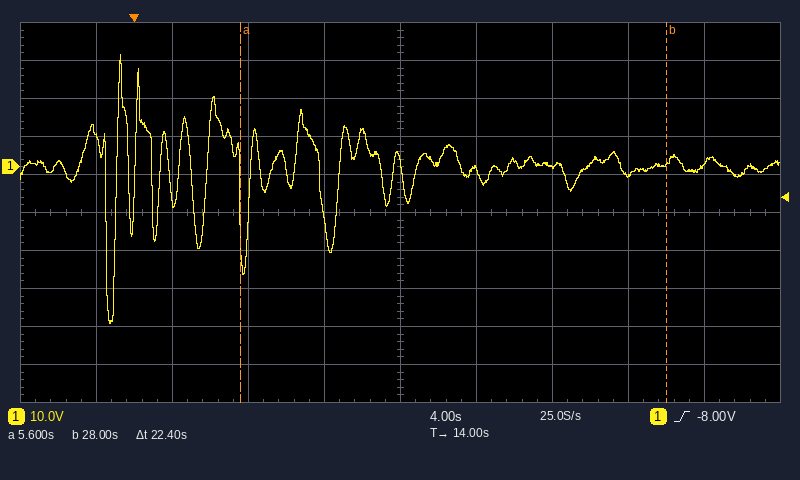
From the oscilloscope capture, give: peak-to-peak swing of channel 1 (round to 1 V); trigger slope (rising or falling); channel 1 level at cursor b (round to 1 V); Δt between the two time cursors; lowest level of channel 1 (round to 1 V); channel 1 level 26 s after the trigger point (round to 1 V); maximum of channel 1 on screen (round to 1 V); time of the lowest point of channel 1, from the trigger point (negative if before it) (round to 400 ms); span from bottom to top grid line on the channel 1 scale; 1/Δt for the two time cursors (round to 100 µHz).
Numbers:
71 V
rising
1 V
22.4 s
-41 V
-2 V
30 V
-1.2 s
100 V
44.6 mHz
